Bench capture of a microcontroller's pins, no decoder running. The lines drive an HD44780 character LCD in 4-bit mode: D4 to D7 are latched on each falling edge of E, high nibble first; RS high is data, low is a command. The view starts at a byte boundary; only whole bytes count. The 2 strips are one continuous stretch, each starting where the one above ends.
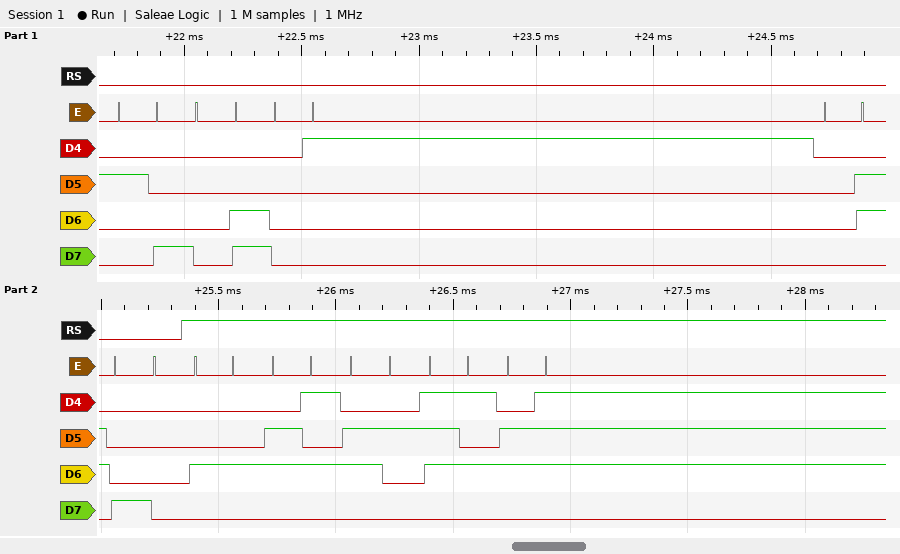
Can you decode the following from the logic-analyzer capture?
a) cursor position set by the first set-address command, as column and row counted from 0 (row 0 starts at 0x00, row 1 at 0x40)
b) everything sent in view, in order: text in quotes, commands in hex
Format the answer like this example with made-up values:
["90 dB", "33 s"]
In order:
["column 0, row 0", "0x28 0x0C 0x01 0x06 0x80 \"Debug\""]
